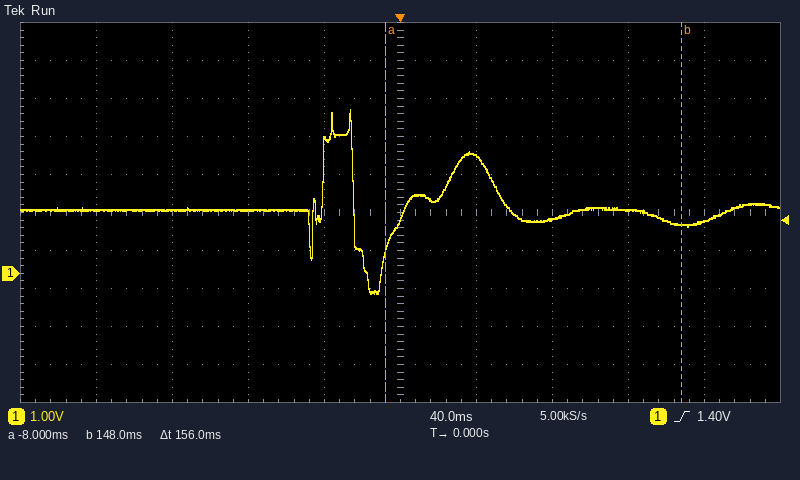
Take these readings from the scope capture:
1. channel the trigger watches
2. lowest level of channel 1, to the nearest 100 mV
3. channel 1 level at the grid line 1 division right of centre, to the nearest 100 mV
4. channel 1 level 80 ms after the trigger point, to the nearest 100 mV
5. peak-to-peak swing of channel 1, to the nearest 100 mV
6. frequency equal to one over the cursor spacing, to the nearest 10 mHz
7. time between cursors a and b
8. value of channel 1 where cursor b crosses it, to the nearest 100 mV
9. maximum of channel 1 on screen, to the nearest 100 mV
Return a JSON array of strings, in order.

["channel 1", "-500 mV", "3.1 V", "1.4 V", "4.8 V", "6.41 Hz", "156 ms", "1.3 V", "4.3 V"]
